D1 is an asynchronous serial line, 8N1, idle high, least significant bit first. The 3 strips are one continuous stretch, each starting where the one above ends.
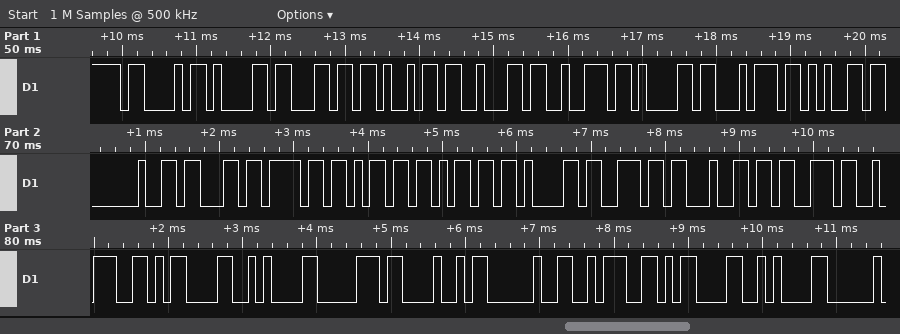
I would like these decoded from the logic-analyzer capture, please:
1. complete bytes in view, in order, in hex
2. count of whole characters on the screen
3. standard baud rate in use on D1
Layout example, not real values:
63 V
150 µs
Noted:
43 61 6C 69 62 72 61 74 65 20 63 6F 6D 6D 61 6E 64 73 3A 0D 0A 70 48 20 3A 0D 0A
27
9600 baud
